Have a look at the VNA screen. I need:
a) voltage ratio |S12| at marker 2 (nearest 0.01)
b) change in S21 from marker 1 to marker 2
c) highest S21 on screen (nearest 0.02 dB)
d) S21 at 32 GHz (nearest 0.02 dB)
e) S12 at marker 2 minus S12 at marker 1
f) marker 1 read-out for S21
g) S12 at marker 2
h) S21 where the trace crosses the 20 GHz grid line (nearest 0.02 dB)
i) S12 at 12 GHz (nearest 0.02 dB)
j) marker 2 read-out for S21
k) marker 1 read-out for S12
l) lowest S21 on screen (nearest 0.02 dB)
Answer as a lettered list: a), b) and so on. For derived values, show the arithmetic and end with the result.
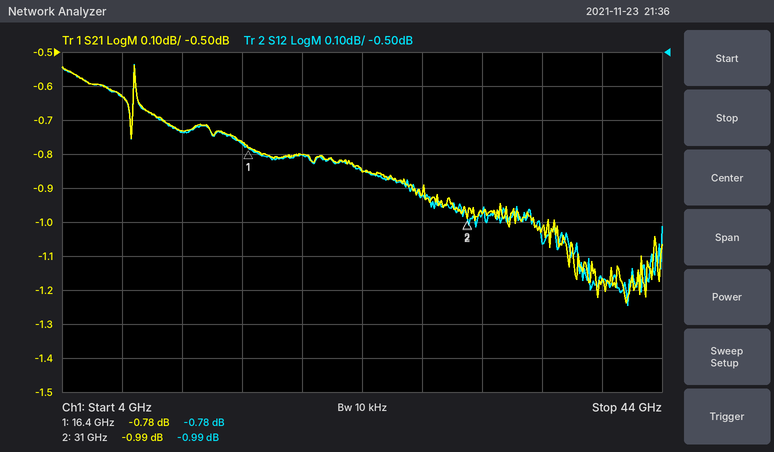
a) 10^(-0.99/20) ≈ 0.89
b) -0.99 − (-0.78) = -0.21 dB
c) -0.54 dB
d) -0.98 dB
e) -0.99 − (-0.78) = -0.21 dB
f) -0.78 dB
g) -0.99 dB
h) -0.80 dB
i) -0.74 dB
j) -0.99 dB
k) -0.78 dB
l) -1.24 dB
